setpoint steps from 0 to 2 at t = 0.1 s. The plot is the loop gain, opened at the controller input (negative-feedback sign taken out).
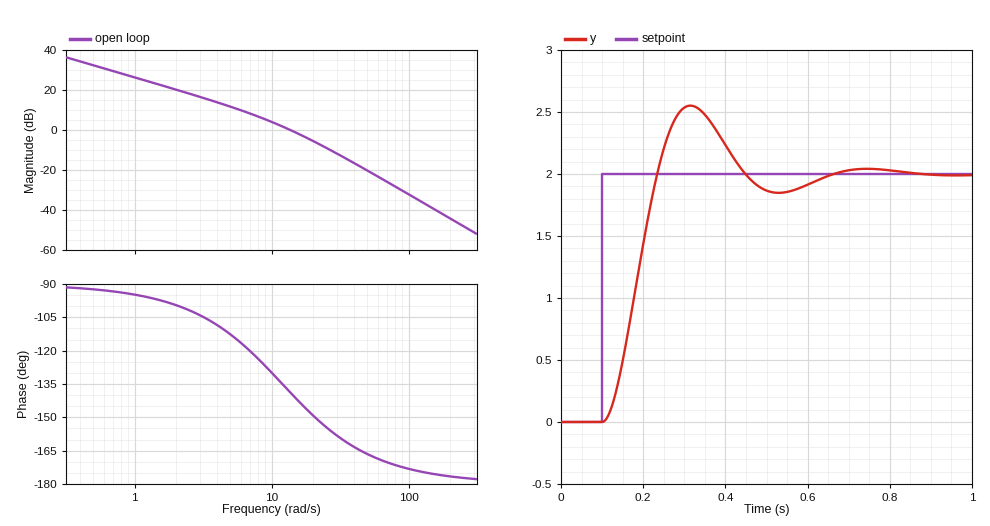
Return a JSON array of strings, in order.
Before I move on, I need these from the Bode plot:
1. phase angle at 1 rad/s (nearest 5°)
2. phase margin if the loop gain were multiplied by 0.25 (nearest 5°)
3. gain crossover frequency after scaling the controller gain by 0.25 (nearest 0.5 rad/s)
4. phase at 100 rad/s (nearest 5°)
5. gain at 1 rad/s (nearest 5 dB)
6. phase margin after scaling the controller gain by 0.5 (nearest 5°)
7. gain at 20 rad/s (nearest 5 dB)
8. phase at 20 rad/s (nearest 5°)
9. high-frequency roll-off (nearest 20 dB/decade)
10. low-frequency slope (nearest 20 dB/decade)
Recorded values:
["-95°", "70°", "5.0 rad/s", "-175°", "25 dB", "55°", "-5 dB", "-150°", "-40 dB/decade", "-20 dB/decade"]
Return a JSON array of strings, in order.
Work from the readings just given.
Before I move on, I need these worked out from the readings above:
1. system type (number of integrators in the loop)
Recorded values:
["1"]
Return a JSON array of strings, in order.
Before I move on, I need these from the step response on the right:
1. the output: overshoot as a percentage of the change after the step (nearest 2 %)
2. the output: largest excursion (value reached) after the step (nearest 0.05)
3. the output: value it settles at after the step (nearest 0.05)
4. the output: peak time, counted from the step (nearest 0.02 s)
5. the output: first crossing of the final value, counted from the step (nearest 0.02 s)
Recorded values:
["28 %", "2.55", "2.00", "0.22 s", "0.14 s"]
